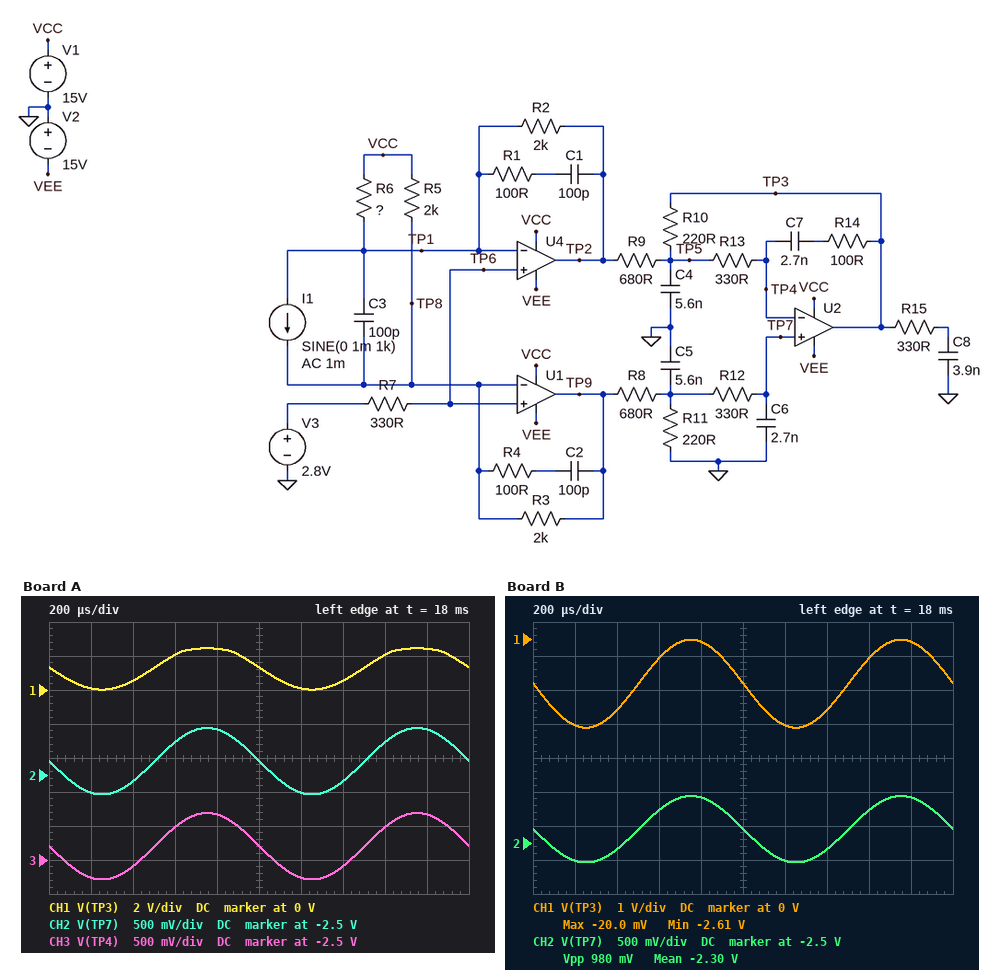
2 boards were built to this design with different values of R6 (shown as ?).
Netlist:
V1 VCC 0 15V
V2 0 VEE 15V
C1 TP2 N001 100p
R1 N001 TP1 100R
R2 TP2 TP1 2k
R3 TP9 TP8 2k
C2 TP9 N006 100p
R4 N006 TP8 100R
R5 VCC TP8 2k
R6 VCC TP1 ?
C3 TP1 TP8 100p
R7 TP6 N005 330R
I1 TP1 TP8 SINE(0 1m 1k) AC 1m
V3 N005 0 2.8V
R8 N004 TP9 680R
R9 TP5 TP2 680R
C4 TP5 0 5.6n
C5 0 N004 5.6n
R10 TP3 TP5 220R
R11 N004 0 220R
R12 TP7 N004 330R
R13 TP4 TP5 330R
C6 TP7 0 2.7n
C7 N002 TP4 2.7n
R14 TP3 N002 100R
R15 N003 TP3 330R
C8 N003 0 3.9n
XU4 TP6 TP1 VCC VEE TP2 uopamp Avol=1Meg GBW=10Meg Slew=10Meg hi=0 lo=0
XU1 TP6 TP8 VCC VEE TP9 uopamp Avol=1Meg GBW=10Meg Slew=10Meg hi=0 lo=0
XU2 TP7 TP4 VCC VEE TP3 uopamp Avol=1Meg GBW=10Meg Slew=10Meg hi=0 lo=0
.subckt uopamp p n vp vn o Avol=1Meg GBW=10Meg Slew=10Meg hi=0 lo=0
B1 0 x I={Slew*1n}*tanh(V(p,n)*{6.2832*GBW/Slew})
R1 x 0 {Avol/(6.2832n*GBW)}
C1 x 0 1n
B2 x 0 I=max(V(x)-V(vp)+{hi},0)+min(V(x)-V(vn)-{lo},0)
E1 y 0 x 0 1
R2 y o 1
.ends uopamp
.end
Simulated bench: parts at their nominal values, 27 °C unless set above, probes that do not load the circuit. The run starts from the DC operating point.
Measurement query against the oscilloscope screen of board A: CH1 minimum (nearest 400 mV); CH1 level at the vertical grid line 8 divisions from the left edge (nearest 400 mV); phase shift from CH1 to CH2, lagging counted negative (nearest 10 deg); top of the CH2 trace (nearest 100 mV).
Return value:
0 V
2.0 V
0 deg
-1.8 V
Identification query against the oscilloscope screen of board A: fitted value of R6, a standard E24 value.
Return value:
1.5 kΩ
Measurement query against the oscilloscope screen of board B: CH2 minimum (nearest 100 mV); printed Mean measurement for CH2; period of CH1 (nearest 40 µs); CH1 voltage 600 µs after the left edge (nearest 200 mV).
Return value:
-2.8 V
-2.30 V
1.00 ms
-600 mV
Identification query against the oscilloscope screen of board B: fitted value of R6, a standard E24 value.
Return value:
3 kΩ
